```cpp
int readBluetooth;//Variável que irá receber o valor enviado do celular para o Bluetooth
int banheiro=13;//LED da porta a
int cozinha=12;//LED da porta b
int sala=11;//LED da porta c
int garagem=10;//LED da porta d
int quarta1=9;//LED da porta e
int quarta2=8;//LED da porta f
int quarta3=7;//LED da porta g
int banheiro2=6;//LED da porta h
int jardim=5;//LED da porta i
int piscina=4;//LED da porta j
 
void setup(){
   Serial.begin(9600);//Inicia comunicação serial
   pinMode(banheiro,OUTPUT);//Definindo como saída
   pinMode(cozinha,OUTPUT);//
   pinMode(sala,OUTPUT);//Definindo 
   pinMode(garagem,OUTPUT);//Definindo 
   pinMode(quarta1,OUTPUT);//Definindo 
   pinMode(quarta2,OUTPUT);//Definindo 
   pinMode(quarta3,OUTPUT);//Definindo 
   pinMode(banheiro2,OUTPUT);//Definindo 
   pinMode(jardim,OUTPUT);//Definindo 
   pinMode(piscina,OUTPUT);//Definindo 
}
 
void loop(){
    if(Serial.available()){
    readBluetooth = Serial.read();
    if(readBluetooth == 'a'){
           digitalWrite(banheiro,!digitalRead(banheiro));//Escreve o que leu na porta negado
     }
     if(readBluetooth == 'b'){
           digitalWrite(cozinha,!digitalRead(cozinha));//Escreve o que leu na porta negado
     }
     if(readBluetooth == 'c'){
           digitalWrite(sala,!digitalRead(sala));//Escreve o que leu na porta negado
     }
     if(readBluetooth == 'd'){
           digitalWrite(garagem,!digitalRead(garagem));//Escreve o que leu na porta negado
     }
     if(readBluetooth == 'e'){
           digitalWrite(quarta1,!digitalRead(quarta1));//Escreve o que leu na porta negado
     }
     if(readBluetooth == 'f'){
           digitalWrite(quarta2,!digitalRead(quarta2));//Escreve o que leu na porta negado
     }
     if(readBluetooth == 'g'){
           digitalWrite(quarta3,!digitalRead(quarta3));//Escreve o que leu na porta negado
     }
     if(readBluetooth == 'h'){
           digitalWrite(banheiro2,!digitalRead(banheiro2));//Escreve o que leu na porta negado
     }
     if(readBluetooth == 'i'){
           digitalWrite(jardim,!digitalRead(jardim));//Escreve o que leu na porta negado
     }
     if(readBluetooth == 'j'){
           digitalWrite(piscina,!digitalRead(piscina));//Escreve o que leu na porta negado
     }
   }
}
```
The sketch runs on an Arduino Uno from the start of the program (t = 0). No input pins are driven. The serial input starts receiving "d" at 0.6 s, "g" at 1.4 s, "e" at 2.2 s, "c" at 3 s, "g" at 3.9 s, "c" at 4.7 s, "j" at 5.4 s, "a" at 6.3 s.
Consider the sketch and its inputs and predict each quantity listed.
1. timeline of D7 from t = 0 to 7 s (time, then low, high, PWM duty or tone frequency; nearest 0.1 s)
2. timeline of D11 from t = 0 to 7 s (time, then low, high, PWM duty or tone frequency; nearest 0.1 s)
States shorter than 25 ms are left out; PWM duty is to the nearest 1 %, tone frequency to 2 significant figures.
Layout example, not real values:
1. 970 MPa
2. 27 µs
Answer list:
1. 0 s low; 1.4 s high; 3.9 s low
2. 0 s low; 3 s high; 4.7 s low
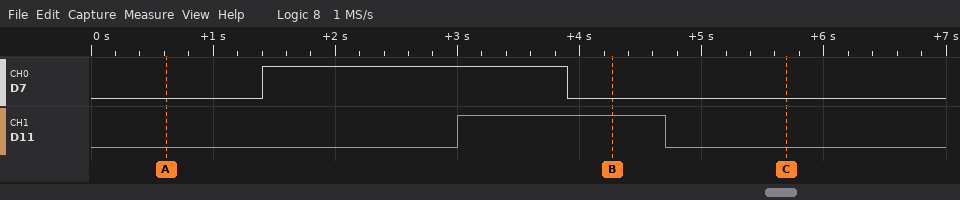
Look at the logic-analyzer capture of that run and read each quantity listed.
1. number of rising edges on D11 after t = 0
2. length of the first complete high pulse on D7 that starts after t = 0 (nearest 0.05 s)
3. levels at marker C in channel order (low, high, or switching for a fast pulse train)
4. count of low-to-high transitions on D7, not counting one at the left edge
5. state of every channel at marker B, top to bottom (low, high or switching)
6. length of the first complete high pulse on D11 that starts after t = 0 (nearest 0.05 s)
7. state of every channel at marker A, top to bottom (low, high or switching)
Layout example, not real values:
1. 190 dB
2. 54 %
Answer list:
1. 1
2. 2.50 s
3. D7 low, D11 low
4. 1
5. D7 low, D11 high
6. 1.70 s
7. D7 low, D11 low
